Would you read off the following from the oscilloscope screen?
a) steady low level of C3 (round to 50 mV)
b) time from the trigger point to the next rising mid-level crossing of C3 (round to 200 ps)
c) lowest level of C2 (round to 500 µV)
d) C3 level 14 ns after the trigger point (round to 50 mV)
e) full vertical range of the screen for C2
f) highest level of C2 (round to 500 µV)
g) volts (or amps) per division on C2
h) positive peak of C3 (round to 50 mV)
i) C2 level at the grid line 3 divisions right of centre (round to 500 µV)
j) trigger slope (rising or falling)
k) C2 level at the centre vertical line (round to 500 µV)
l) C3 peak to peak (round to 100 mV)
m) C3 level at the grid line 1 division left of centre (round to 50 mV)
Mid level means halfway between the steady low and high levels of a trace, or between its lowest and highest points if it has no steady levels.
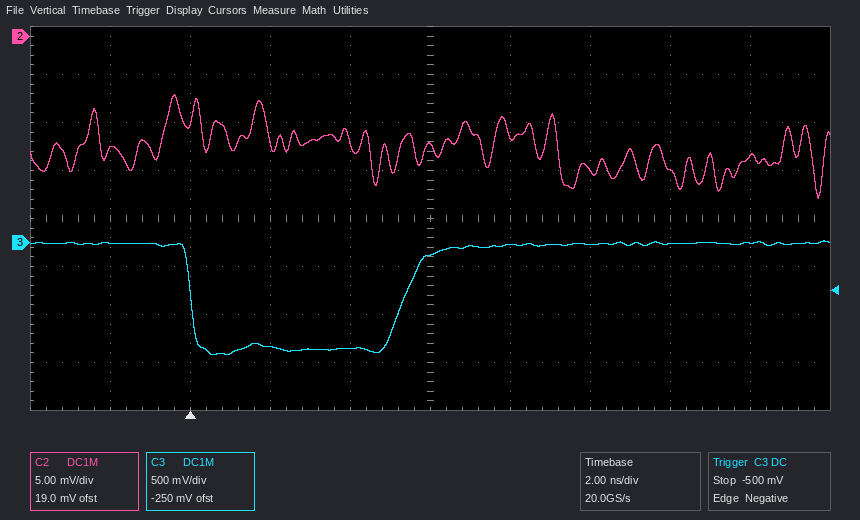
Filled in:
-1.10 V
5.4 ns
-17.0 mV
0 mV
40 mV
-6.0 mV
5 mV
0 mV
-14.0 mV
falling
-11.5 mV
1.20 V
-1.10 V
